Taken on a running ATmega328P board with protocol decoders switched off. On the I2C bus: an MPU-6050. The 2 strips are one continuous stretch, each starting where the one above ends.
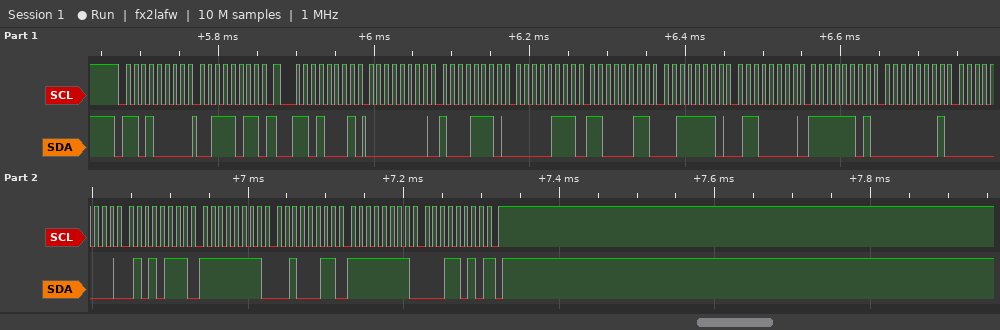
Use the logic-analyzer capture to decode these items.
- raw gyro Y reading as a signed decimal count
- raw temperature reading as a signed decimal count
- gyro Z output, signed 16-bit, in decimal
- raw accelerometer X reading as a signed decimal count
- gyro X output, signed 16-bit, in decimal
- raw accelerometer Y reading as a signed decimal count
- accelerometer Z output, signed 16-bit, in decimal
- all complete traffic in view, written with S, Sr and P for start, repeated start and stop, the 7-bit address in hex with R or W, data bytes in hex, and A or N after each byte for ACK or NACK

-221
-767
-230
142
87
1987
15968
S 68W A 3B A Sr 68R A 00 A 8E A 07 A C3 A 3E A 60 A FD A 01 A 00 A 57 A FF A 23 A FF A 1A N P
